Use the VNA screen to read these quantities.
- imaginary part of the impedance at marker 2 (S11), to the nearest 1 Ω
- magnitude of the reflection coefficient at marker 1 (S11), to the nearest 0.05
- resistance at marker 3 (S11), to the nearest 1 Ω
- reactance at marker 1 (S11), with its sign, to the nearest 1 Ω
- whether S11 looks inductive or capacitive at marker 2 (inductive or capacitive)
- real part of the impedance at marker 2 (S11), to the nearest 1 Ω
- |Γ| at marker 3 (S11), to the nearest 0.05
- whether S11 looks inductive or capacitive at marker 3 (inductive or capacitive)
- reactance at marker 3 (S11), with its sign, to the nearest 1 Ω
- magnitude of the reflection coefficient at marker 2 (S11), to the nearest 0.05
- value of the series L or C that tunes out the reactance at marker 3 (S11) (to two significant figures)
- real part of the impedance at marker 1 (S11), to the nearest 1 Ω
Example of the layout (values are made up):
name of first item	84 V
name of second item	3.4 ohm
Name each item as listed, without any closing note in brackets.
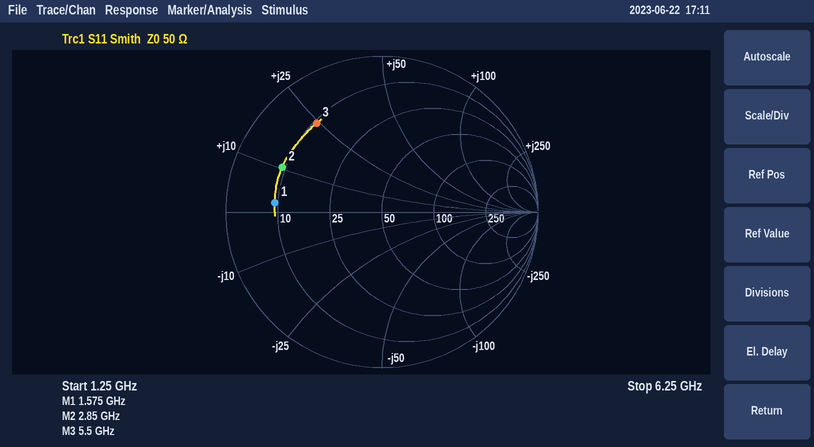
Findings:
imaginary part of the impedance at marker 2 (S11), to the nearest 1 Ω	+10 Ω
magnitude of the reflection coefficient at marker 1 (S11), to the nearest 0.05	0.70
resistance at marker 3 (S11), to the nearest 1 Ω	11 Ω
reactance at marker 1 (S11), with its sign, to the nearest 1 Ω	+2 Ω
whether S11 looks inductive or capacitive at marker 2	inductive
real part of the impedance at marker 2 (S11), to the nearest 1 Ω	9 Ω
|Γ| at marker 3 (S11), to the nearest 0.05	0.70
whether S11 looks inductive or capacitive at marker 3	inductive
reactance at marker 3 (S11), with its sign, to the nearest 1 Ω	+24 Ω
magnitude of the reflection coefficient at marker 2 (S11), to the nearest 0.05	0.70
value of the series L or C that tunes out the reactance at marker 3 (S11)	1.2 pF
real part of the impedance at marker 1 (S11), to the nearest 1 Ω	9 Ω
